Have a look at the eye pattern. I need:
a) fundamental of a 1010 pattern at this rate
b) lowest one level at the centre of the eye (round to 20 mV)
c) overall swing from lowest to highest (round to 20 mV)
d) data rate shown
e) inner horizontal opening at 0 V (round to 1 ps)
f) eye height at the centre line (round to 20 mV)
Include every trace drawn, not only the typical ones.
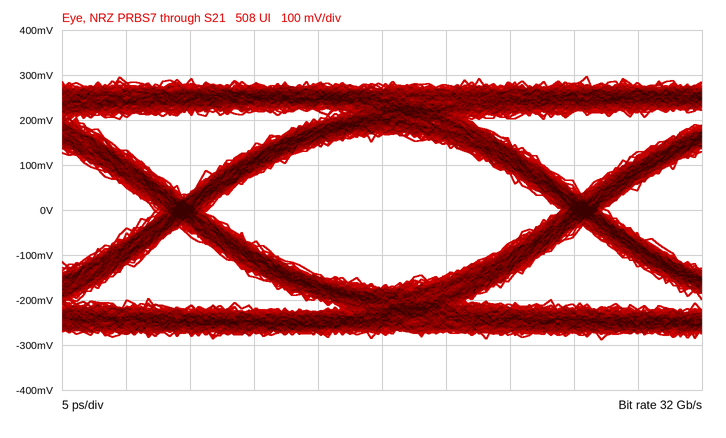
16 GHz
160 mV
580 mV
32 Gb/s
28 ps
340 mV
